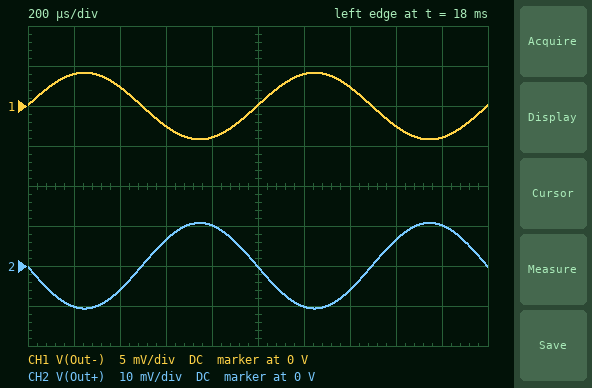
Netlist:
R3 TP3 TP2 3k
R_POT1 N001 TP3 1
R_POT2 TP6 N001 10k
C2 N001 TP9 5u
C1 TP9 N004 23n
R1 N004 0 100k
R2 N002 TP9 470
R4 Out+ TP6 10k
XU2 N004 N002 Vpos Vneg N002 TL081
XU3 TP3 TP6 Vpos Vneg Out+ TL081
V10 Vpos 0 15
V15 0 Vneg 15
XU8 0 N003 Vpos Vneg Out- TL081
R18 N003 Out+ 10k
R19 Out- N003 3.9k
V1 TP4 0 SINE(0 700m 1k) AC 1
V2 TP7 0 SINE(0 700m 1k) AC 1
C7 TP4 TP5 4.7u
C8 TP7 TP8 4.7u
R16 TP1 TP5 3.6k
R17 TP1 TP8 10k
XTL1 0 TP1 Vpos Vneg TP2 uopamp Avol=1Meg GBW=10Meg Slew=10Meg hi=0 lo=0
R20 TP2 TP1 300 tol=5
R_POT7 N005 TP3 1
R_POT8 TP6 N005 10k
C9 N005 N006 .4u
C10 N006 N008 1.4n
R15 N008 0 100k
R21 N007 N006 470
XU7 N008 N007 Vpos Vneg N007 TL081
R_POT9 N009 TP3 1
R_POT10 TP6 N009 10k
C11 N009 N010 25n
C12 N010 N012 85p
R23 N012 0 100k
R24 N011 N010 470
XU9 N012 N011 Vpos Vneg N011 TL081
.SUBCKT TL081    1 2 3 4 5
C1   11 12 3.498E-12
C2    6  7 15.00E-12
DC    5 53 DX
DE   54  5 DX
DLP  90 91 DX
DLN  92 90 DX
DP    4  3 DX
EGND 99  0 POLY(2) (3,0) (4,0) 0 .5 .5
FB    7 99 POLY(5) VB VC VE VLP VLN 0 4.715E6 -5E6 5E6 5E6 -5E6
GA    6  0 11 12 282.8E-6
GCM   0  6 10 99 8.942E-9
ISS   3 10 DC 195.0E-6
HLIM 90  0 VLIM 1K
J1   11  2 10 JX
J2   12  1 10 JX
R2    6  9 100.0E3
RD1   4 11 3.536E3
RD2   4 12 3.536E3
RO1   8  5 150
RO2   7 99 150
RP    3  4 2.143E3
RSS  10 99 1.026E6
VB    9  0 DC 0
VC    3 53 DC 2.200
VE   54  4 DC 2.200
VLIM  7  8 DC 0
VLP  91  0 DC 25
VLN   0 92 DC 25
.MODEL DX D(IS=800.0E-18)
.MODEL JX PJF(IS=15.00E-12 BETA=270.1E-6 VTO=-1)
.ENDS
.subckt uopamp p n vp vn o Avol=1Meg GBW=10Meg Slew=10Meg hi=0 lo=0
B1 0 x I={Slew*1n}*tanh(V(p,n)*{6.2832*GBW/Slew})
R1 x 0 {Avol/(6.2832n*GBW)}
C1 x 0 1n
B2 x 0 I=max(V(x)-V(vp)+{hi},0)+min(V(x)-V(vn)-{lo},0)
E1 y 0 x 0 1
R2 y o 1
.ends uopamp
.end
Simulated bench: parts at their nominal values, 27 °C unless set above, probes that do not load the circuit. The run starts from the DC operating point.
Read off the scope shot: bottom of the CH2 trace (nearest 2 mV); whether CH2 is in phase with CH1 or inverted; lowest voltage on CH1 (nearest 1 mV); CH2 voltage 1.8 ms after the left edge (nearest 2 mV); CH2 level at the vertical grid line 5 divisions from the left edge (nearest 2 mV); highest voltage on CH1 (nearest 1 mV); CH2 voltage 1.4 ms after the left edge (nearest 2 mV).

-10 mV
inverted
-4 mV
10 mV
0 V
4 mV
-6 mV
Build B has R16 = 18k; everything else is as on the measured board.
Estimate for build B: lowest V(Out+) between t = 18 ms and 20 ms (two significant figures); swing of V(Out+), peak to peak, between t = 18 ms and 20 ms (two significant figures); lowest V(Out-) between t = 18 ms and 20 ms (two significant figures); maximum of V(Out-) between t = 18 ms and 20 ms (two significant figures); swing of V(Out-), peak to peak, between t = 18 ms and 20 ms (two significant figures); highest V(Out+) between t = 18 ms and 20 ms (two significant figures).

-4.4 mV
8.8 mV
-1.7 mV
1.7 mV
3.4 mV
4.4 mV
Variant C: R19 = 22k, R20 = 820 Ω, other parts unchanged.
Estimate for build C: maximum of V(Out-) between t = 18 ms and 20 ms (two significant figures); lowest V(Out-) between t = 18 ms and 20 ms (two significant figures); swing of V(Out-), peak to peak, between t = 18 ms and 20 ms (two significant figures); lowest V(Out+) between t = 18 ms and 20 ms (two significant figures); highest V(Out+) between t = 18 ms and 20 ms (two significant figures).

64 mV
-64 mV
130 mV
-29 mV
29 mV
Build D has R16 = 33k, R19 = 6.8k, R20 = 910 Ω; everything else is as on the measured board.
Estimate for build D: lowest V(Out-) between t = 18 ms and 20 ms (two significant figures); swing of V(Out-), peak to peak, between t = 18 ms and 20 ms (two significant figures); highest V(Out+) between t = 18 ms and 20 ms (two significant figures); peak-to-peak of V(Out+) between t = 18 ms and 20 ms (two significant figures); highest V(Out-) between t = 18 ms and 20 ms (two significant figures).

-7.6 mV
15 mV
11 mV
22 mV
7.7 mV
